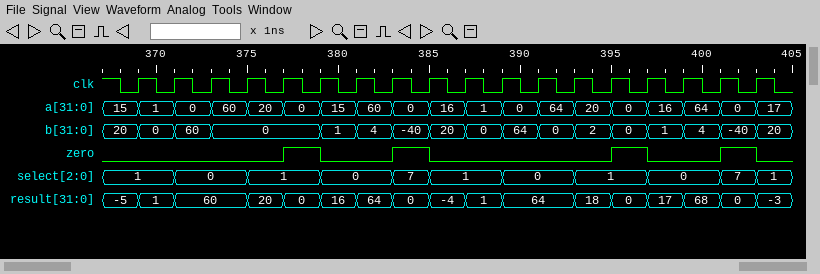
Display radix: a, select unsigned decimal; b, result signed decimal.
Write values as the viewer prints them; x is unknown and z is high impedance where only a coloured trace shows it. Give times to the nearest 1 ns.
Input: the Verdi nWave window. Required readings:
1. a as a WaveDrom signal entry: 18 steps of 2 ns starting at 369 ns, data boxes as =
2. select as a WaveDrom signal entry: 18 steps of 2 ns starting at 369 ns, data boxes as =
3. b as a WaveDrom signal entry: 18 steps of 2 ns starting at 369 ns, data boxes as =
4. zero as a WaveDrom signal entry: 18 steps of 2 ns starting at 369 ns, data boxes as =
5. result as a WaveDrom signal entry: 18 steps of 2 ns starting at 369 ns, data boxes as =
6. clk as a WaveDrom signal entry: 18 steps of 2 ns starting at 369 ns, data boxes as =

{name: 'a', wave: '==================', data: '1 0 60 20 0 15 60 0 16 1 0 64 20 0 16 64 0 17'}
{name: 'select', wave: '==.=.=.==.=.=.=.==', data: '1 0 1 0 7 1 0 1 0 7 1'}
{name: 'b', wave: '===..=============', data: '0 60 0 1 4 -40 20 0 64 0 2 0 1 4 -40 20'}
{name: 'zero', wave: '0...10.10....10.10'}
{name: 'result', wave: '==.========.======', data: '1 60 20 0 16 64 0 -4 1 64 18 0 17 68 0 -3'}
{name: 'clk', wave: 'p.................'}
